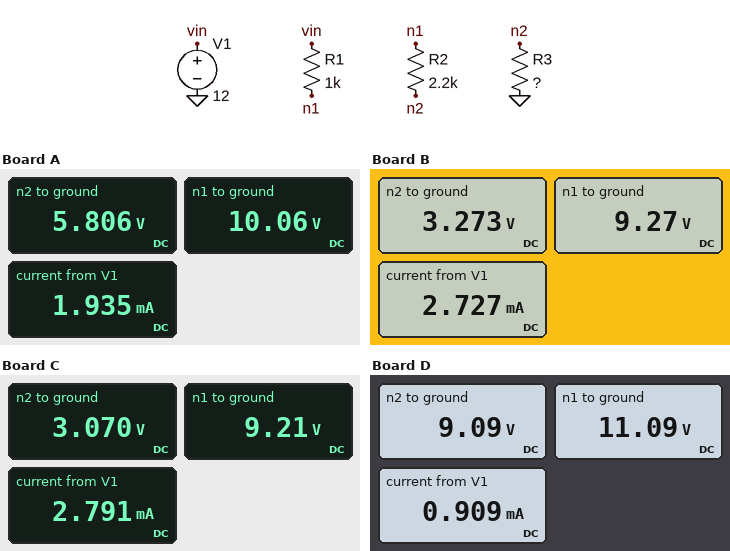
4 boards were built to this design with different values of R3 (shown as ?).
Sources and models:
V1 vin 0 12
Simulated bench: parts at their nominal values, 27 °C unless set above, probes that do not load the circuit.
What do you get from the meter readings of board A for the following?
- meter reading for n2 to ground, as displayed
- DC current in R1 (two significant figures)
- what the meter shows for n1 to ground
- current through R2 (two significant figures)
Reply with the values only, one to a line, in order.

5.806 V
1.9 mA
10.06 V
1.9 mA
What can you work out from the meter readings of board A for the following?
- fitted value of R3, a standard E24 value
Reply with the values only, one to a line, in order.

3 kΩ
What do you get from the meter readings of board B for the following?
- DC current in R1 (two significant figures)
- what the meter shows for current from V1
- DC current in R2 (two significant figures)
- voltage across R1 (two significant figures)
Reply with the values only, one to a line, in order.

2.7 mA
2.727 mA
2.7 mA
2.7 V
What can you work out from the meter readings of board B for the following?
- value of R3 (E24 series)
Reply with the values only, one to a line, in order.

1.2 kΩ
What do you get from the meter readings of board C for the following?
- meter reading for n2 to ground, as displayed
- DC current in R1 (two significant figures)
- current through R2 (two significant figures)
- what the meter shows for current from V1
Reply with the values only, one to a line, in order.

3.070 V
2.8 mA
2.8 mA
2.791 mA
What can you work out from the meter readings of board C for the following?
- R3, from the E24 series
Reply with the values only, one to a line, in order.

1.1 kΩ
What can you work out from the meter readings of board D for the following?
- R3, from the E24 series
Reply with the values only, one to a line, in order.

10 kΩ
